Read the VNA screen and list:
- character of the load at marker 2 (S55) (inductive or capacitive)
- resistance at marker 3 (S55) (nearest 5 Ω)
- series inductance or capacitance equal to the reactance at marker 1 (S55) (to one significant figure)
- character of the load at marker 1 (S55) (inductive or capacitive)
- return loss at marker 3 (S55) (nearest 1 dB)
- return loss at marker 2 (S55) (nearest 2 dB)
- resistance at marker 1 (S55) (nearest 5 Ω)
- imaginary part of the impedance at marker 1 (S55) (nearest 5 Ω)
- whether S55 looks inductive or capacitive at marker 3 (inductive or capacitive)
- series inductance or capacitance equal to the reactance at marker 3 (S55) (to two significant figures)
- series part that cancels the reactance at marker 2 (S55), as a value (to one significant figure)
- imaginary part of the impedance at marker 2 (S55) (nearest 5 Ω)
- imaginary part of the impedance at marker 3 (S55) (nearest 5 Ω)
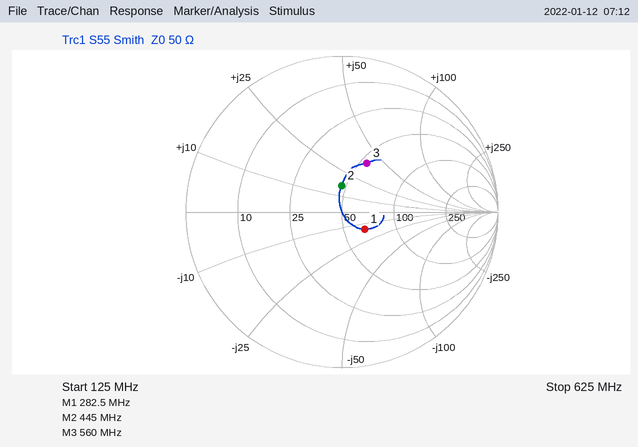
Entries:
inductive
55 Ω
40 pF
capacitive
9 dB
16 dB
65 Ω
-15 Ω
inductive
11 nH
20 pF
+15 Ω
+40 Ω
